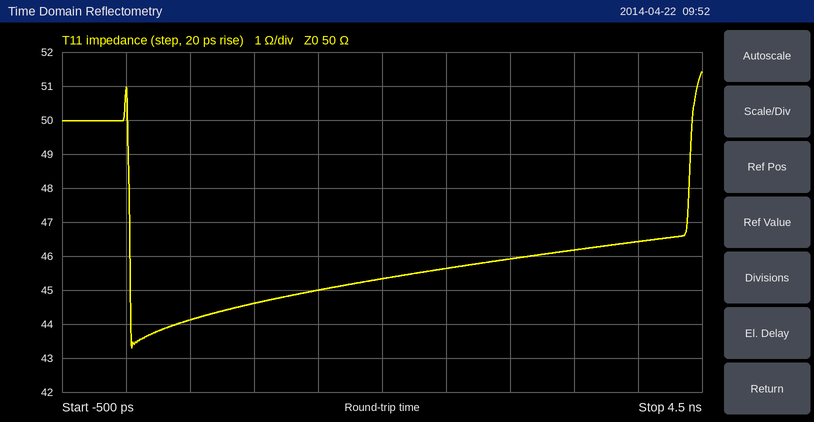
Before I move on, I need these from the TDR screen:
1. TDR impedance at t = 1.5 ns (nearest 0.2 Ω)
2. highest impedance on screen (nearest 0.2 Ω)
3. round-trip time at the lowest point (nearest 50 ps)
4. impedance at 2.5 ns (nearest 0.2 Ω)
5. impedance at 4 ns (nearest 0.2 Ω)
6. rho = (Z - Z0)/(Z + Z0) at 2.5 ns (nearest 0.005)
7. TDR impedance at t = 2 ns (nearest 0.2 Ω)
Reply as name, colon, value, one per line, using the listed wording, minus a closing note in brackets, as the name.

TDR impedance at t = 1.5 ns: 45.0 Ω
highest impedance on screen: 51.4 Ω
round-trip time at the lowest point: 50 ps
impedance at 2.5 ns: 45.6 Ω
impedance at 4 ns: 46.4 Ω
rho = (Z - Z0)/(Z + Z0) at 2.5 ns: -0.045
TDR impedance at t = 2 ns: 45.4 Ω
